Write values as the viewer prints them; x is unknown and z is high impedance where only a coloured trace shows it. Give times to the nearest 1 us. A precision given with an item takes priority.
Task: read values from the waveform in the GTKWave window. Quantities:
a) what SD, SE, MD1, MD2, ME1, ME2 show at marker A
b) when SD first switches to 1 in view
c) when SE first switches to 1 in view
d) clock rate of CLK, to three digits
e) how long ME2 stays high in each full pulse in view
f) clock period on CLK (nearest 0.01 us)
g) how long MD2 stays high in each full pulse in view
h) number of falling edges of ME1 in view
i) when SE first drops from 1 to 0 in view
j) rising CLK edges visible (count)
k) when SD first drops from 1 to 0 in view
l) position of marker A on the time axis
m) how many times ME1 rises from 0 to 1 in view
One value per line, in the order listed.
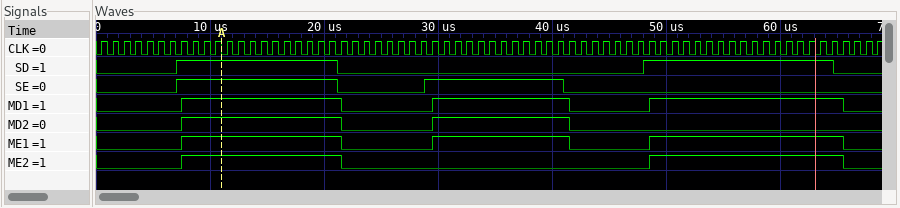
SD=1, SE=1, MD1=1, MD2=1, ME1=1, ME2=1
7 us
7 us
1.00 MHz
14 us, 17 us
1 us
14 us, 12 us
3
21 us
69
21 us
11 us
3
